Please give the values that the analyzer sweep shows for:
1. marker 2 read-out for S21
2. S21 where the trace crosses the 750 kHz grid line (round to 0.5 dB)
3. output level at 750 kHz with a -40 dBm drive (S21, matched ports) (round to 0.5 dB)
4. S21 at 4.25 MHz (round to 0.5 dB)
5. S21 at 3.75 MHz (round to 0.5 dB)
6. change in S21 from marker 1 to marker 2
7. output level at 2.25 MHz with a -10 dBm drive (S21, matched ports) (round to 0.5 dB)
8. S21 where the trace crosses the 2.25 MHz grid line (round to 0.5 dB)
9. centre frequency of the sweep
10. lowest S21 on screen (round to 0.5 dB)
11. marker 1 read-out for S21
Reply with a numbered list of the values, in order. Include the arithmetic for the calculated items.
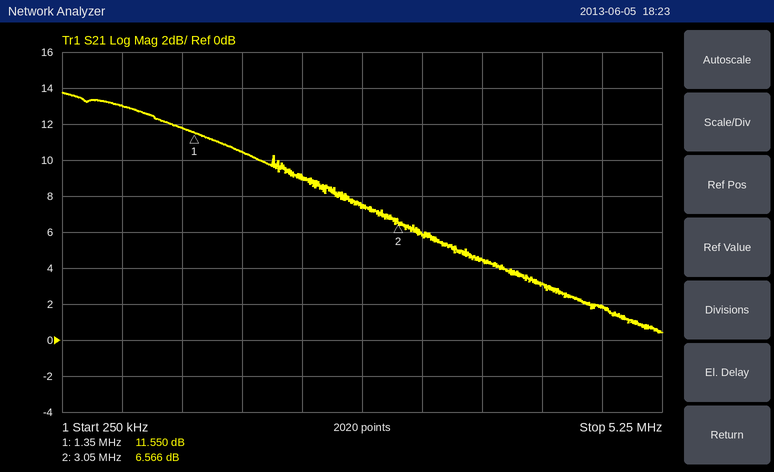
1. 6.566 dB
2. 13.0 dB
3. -40 dBm + (13.0 dB) = -27.0 dBm
4. 3.0 dB
5. 4.5 dB
6. 6.566 − (11.55) = -4.984 dB
7. -10 dBm + (9.0 dB) = -1.0 dBm
8. 9.0 dB
9. 2.75 MHz
10. 0.5 dB
11. 11.550 dB
